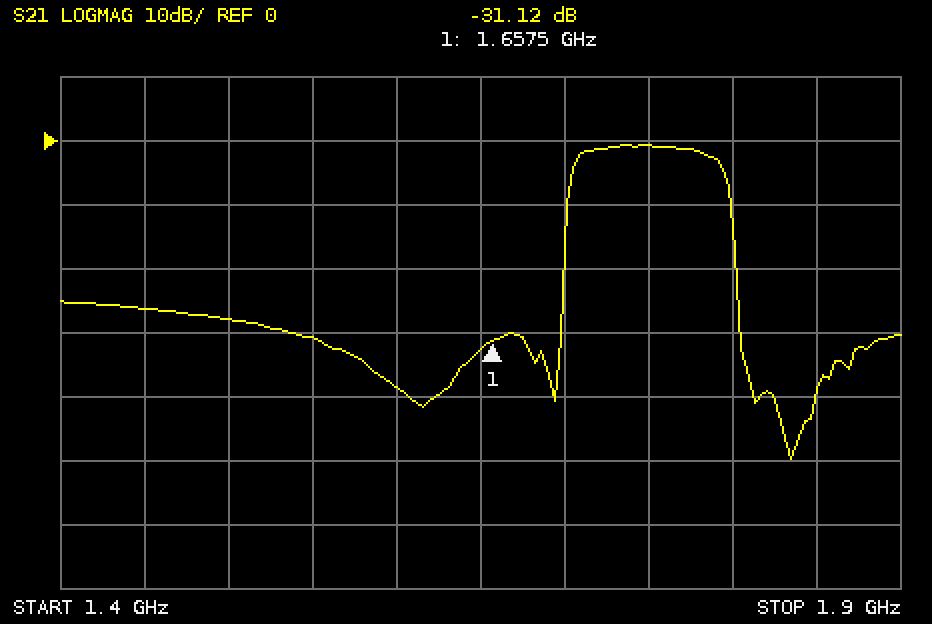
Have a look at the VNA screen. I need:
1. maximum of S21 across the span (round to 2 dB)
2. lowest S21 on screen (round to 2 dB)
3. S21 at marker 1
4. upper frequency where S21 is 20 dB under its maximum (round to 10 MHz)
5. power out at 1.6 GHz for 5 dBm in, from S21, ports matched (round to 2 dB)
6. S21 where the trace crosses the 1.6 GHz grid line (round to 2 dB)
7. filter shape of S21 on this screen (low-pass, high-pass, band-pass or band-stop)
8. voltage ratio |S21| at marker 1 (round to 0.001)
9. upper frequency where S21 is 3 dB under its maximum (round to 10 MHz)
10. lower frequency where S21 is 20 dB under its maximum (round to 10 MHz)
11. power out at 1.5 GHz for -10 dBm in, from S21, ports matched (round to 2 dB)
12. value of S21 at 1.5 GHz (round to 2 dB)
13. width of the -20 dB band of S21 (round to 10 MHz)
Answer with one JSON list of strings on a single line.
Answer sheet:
["0 dB", "-50 dB", "-31.12 dB", "1.80 GHz", "-34 dBm", "-38 dB", "band-pass", "0.028", "1.79 GHz", "1.70 GHz", "-38 dBm", "-28 dB", "100 MHz"]
